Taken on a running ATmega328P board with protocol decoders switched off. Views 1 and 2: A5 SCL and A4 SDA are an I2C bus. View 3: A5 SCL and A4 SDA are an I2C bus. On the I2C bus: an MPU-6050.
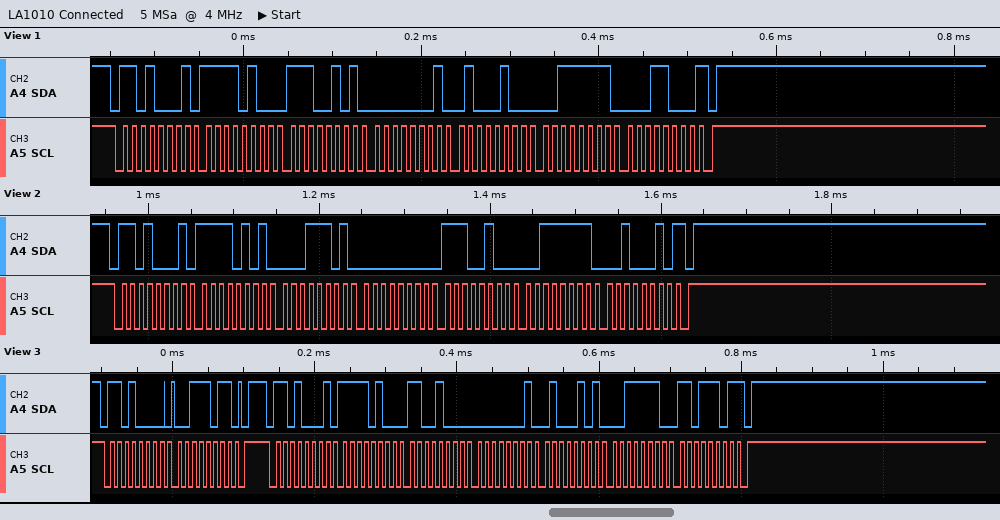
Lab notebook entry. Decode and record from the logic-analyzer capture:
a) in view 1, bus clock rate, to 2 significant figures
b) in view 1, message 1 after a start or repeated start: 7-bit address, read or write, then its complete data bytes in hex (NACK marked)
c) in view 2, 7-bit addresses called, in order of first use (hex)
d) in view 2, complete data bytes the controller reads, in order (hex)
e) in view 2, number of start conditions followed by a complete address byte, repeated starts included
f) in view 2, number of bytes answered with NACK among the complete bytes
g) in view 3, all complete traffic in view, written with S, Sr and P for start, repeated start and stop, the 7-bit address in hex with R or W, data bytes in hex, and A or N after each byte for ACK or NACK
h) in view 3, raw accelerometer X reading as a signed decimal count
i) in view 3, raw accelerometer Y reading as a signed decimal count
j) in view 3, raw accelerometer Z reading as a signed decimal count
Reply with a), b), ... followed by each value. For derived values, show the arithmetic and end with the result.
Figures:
a) 100 kHz
b) 0x68 read: F4 E5 01 44 3F 18 NACK
c) 0x68
d) F5 1D 00 E4 3F 22
e) 1
f) 1
g) S 68W A 3B A P S 68R A F4 A C8 A 01 A 45 A 3E A DD N P
h) 0xF4C8 = -2872
i) 0x0145 = 325
j) 0x3EDD = 16093
